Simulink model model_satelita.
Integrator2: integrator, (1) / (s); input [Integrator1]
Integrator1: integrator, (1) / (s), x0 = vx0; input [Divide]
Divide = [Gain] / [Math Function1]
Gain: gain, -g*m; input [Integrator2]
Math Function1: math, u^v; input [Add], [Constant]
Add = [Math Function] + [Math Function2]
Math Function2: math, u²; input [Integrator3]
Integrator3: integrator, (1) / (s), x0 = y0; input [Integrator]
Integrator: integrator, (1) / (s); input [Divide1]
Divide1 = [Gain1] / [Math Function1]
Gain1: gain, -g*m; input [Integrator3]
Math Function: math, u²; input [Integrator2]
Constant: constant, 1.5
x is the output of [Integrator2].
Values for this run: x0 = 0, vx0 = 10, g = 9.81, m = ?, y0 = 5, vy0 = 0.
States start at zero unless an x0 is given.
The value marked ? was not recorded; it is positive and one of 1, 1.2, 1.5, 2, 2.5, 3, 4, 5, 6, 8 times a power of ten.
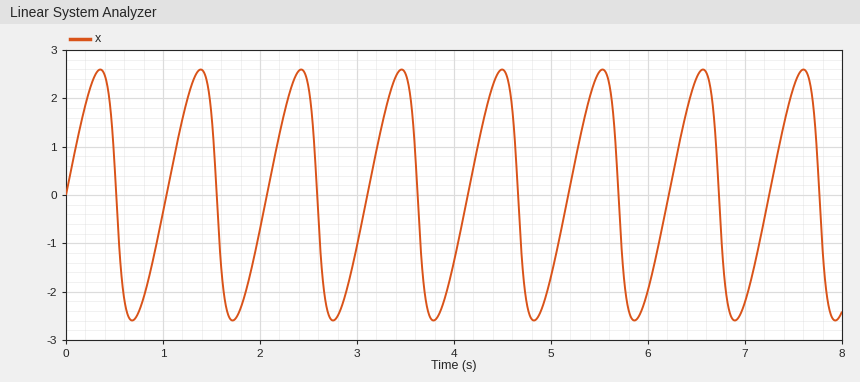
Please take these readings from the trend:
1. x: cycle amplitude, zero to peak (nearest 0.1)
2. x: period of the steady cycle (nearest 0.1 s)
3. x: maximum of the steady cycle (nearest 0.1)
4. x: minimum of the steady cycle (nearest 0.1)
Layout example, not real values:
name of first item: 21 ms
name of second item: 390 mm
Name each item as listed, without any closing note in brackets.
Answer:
x: cycle amplitude, zero to peak: 2.6
x: period of the steady cycle: 1.0 s
x: maximum of the steady cycle: 2.6
x: minimum of the steady cycle: -2.6
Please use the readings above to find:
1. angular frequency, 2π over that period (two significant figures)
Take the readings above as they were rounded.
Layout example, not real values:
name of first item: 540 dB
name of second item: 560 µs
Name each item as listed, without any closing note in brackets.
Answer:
angular frequency, 2π over that period: 6.3 rad/s
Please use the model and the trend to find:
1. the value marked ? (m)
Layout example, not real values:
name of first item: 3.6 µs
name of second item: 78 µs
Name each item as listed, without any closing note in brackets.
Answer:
the value marked ?: 120
